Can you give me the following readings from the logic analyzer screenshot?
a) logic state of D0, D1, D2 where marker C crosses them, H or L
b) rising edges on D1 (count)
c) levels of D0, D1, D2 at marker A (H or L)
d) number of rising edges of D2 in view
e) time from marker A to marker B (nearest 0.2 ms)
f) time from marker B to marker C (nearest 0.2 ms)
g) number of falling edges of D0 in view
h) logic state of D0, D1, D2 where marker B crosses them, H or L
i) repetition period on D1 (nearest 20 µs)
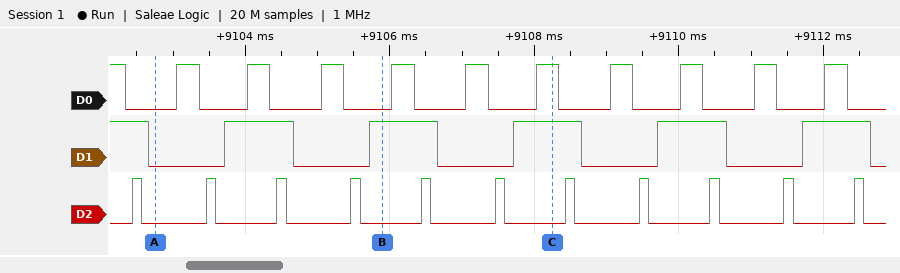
D0=H, D1=H, D2=L
5
D0=L, D1=L, D2=L
11
3.2 ms
2.4 ms
11
D0=L, D1=H, D2=L
2000 µs
